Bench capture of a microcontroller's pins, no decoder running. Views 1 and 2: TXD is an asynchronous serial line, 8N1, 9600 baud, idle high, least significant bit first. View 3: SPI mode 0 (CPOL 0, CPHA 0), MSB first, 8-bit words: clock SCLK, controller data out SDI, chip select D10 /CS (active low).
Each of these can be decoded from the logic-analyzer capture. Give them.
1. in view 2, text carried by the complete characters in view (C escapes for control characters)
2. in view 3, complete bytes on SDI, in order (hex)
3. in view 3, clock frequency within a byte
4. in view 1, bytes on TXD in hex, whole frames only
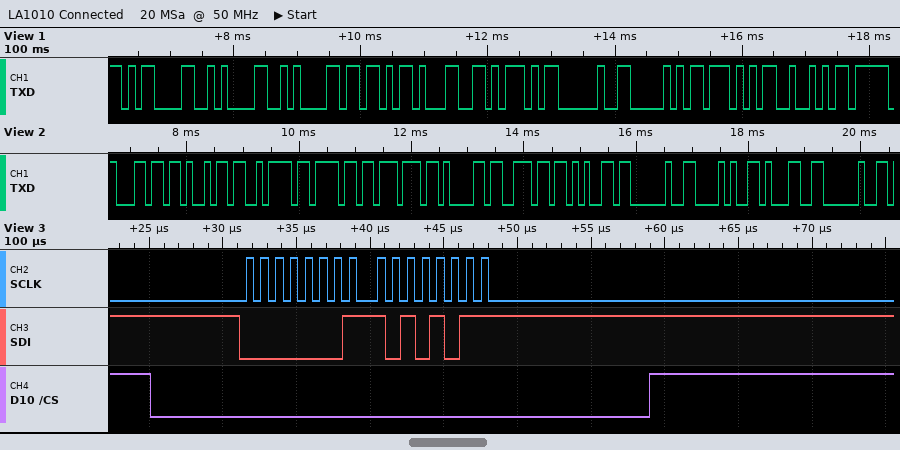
"lizowane (1 "
01 AB
1 MHz
0D 0A 0A 5B 31 5D 20 50 57 52
